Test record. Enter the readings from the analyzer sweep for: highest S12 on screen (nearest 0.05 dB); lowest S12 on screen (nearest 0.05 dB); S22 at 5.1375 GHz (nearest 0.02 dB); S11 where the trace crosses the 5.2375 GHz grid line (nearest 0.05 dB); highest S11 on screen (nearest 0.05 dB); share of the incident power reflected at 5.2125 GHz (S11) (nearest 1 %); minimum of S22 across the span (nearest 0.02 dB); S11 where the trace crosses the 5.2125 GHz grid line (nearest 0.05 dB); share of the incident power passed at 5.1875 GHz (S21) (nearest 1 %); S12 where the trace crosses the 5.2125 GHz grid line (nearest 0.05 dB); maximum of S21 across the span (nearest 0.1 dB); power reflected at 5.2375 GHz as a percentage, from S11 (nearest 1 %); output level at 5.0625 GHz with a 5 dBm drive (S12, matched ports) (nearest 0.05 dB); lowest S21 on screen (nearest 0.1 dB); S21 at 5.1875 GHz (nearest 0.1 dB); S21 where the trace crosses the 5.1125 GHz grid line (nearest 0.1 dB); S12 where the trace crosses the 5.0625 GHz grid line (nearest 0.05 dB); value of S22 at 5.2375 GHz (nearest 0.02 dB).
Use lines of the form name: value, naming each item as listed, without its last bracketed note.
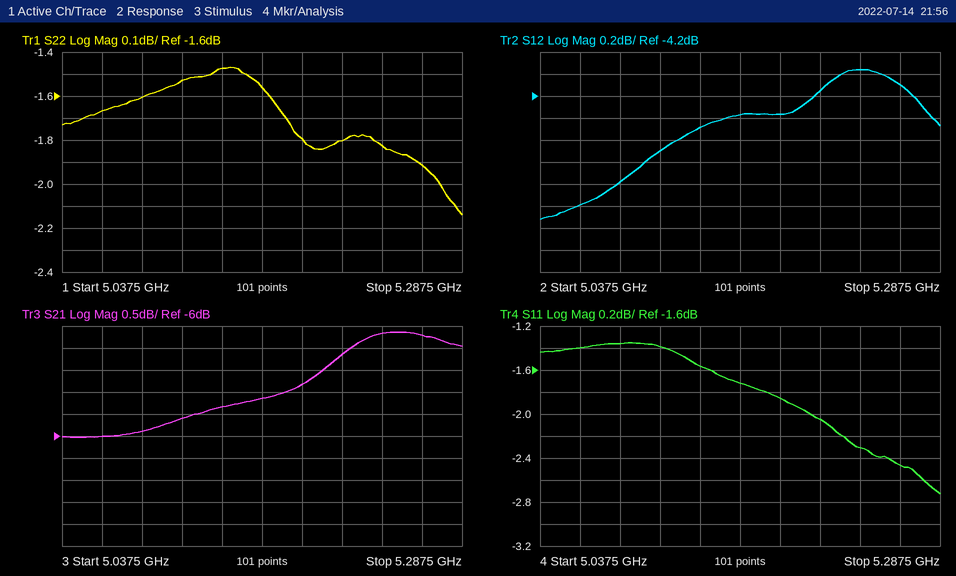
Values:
highest S12 on screen: -3.95 dB
lowest S12 on screen: -5.30 dB
S22 at 5.1375 GHz: -1.48 dB
S11 where the trace crosses the 5.2375 GHz grid line: -2.30 dB
highest S11 on screen: -1.35 dB
share of the incident power reflected at 5.2125 GHz (S11): 62 %
minimum of S22 across the span: -2.14 dB
S11 where the trace crosses the 5.2125 GHz grid line: -2.05 dB
share of the incident power passed at 5.1875 GHz (S21): 33 %
S12 where the trace crosses the 5.2125 GHz grid line: -4.15 dB
maximum of S21 across the span: -3.6 dB
power reflected at 5.2375 GHz as a percentage, from S11: 59 %
output level at 5.0625 GHz with a 5 dBm drive (S12, matched ports): -0.20 dBm
lowest S21 on screen: -6.0 dB
S21 at 5.1875 GHz: -4.8 dB
S21 where the trace crosses the 5.1125 GHz grid line: -5.6 dB
S12 where the trace crosses the 5.0625 GHz grid line: -5.20 dB
value of S22 at 5.2375 GHz: -1.82 dB
